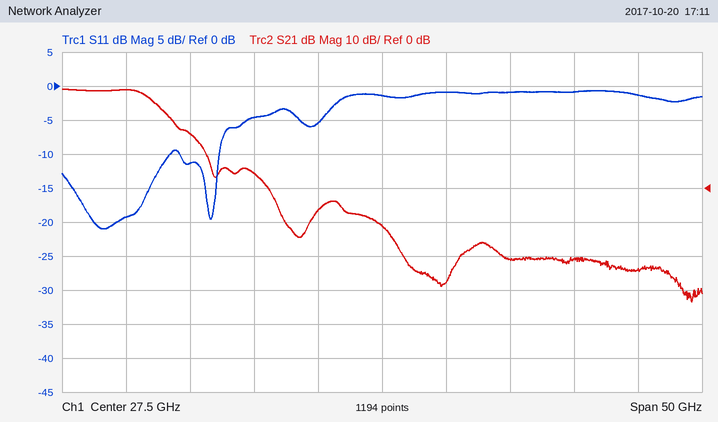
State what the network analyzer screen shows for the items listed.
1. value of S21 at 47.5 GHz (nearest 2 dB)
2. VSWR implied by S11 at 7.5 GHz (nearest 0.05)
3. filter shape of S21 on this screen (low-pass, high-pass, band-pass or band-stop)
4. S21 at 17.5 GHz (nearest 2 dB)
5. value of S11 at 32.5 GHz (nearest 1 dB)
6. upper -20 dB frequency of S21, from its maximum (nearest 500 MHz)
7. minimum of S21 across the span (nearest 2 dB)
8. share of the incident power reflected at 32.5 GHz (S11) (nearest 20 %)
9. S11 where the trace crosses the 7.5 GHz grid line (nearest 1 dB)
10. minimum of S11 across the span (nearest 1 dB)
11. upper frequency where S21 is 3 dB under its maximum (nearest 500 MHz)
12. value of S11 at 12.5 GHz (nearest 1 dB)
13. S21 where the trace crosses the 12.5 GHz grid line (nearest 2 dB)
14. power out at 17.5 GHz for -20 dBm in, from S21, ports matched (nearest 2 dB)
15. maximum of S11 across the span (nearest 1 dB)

-24 dB
1.25
low-pass
4 dB
-1 dB
14.0 GHz
-34 dB
80 %
-19 dB
-21 dB
9.5 GHz
-11 dB
16 dB
-16 dBm
-1 dB
